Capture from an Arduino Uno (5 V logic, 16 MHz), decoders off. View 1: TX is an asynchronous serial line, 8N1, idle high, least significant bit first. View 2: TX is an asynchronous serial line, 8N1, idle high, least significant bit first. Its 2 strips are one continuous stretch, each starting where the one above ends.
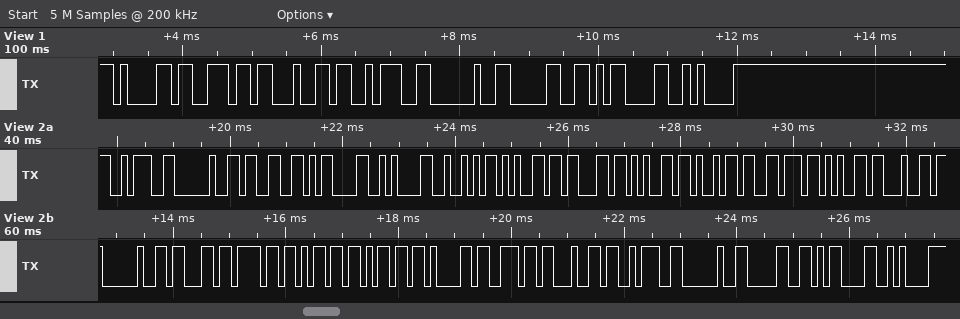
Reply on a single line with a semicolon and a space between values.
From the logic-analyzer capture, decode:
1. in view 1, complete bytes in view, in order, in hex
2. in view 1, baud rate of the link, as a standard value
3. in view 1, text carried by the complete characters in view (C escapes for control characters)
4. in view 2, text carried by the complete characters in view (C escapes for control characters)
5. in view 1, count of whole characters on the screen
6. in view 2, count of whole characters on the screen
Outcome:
61 6E 64 3A 20 30 0D 0A; 9600 baud; "and: 0\r\n"; ": 3\r\nReceived command: 0\r\n"; 8; 26
